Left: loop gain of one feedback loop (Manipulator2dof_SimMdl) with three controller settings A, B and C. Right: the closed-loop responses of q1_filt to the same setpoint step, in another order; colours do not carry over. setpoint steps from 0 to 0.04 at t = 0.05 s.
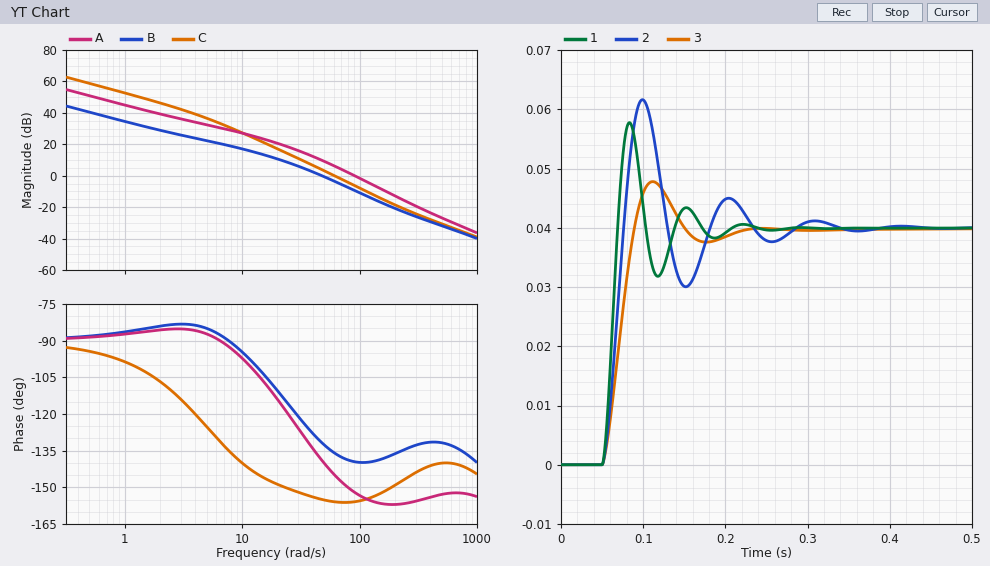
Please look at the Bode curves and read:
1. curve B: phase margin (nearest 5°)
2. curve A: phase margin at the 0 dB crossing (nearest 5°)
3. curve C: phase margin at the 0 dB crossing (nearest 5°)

50°
30°
25°
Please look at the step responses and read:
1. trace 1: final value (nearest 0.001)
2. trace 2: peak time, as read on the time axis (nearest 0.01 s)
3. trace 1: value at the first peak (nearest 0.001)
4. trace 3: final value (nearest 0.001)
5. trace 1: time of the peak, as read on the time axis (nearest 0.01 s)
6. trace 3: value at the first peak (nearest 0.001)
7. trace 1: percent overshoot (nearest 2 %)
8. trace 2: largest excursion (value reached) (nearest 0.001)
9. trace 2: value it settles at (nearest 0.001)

0.040
0.10 s
0.058
0.040
0.08 s
0.048
44 %
0.062
0.040
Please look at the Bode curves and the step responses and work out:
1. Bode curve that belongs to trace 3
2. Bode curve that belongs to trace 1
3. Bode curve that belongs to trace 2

B
A
C
